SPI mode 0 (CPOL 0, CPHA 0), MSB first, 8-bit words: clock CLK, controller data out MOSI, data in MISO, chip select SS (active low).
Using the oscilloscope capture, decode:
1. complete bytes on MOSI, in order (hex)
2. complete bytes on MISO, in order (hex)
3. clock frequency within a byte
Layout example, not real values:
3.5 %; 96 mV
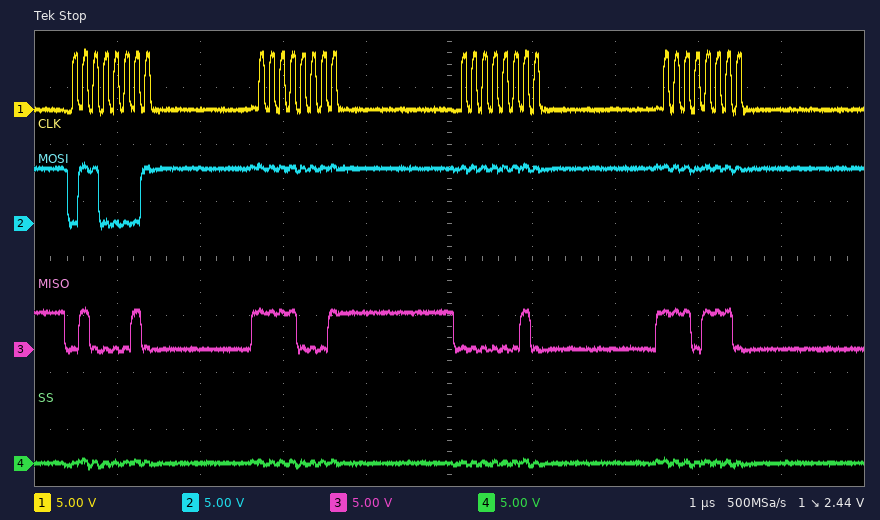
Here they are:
61 FF FF FF; 42 F1 02 EE; 8 MHz
